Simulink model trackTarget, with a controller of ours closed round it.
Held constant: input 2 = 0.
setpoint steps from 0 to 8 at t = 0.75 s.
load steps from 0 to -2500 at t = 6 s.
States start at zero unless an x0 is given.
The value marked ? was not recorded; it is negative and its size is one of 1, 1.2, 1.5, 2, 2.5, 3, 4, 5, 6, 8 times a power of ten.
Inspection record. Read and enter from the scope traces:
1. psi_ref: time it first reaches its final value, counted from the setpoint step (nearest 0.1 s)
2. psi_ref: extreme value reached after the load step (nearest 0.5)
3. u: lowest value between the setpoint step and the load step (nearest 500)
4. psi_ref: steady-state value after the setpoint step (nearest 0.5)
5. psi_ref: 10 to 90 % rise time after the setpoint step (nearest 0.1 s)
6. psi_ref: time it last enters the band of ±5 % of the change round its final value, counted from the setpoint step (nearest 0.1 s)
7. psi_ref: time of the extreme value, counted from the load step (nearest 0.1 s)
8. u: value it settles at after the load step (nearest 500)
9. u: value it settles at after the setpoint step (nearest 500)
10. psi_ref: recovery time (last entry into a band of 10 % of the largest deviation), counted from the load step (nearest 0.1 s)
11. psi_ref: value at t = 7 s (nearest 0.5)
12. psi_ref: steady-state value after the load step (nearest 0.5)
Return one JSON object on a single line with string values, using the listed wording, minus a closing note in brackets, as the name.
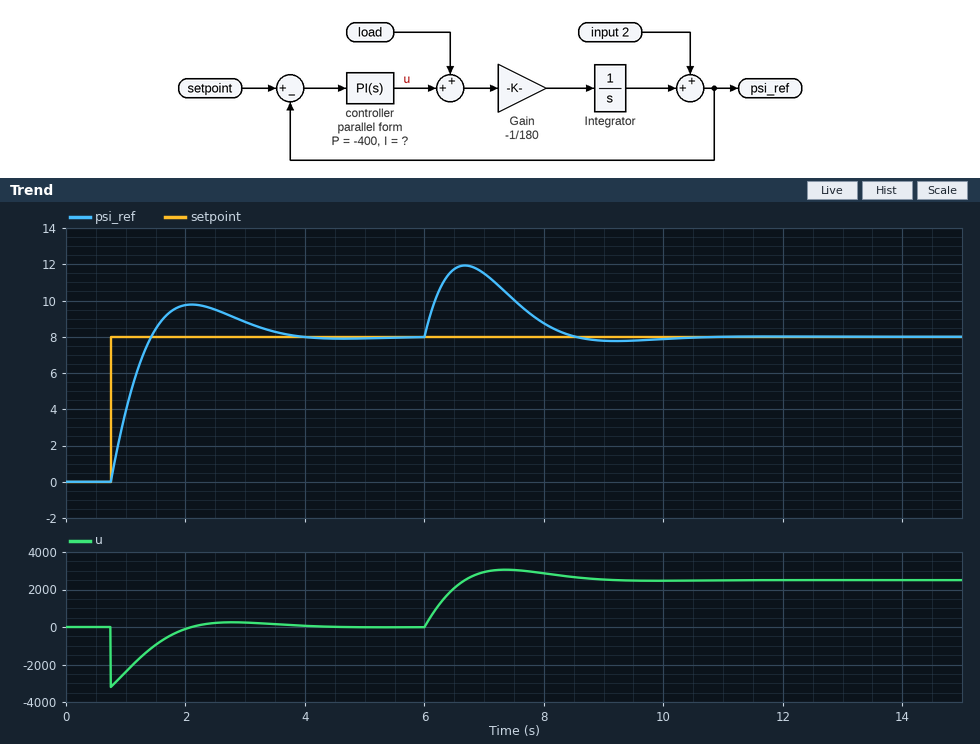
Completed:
{"psi_ref: time it first reaches its final value, counted from the setpoint step": "0.7 s", "psi_ref: extreme value reached after the load step": "12.0", "u: lowest value between the setpoint step and the load step": "-3000", "psi_ref: steady-state value after the setpoint step": "8.0", "psi_ref: 10 to 90 % rise time after the setpoint step": "0.5 s", "psi_ref: time it last enters the band of ±5 % of the change round its final value, counted from the setpoint step": "2.6 s", "psi_ref: time of the extreme value, counted from the load step": "0.7 s", "u: value it settles at after the load step": "2500", "u: value it settles at after the setpoint step": "0", "psi_ref: recovery time (last entry into a band of 10 % of the largest deviation), counted from the load step": "2.2 s", "psi_ref: value at t = 7 s": "11.5", "psi_ref: steady-state value after the load step": "8.0"}
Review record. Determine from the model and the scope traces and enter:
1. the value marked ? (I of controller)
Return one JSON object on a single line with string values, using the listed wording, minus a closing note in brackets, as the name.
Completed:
{"the value marked ?": "-500"}
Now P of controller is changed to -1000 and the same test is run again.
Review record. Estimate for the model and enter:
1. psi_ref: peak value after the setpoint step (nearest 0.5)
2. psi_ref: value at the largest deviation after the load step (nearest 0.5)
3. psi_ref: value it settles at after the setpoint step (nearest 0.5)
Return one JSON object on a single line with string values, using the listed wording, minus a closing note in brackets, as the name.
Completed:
{"psi_ref: peak value after the setpoint step": "8.5", "psi_ref: value at the largest deviation after the load step": "10.0", "psi_ref: value it settles at after the setpoint step": "8.0"}
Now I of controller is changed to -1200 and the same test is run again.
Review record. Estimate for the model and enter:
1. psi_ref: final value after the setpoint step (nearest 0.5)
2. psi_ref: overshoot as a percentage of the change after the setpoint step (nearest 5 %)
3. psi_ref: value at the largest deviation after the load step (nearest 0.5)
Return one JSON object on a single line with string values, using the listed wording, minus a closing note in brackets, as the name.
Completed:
{"psi_ref: final value after the setpoint step": "8.0", "psi_ref: overshoot as a percentage of the change after the setpoint step": "35 %", "psi_ref: value at the largest deviation after the load step": "11.0"}
